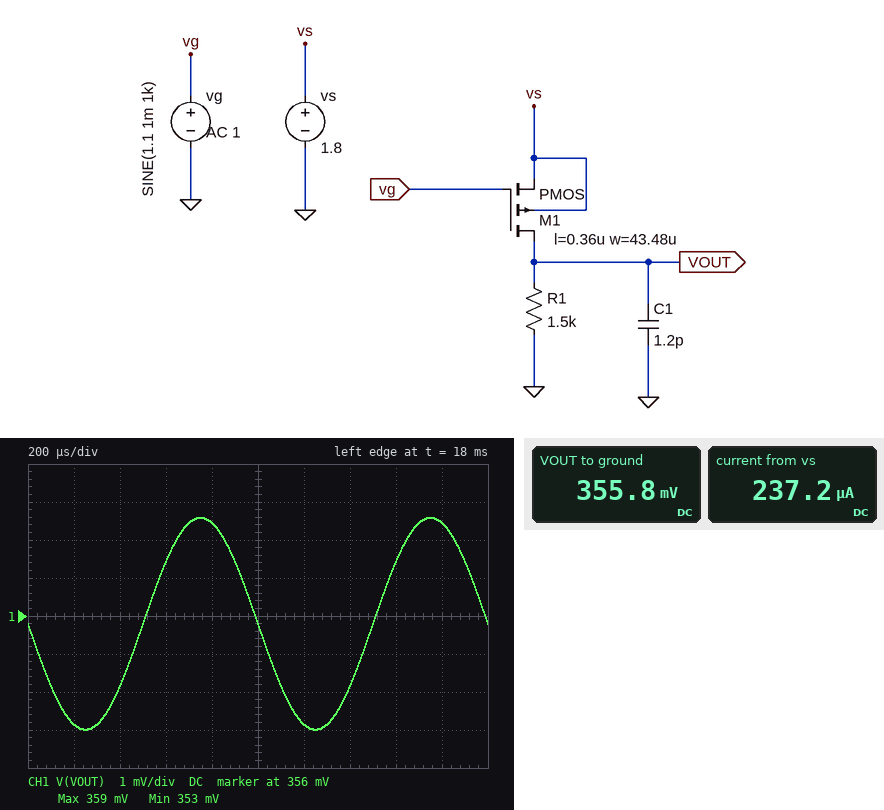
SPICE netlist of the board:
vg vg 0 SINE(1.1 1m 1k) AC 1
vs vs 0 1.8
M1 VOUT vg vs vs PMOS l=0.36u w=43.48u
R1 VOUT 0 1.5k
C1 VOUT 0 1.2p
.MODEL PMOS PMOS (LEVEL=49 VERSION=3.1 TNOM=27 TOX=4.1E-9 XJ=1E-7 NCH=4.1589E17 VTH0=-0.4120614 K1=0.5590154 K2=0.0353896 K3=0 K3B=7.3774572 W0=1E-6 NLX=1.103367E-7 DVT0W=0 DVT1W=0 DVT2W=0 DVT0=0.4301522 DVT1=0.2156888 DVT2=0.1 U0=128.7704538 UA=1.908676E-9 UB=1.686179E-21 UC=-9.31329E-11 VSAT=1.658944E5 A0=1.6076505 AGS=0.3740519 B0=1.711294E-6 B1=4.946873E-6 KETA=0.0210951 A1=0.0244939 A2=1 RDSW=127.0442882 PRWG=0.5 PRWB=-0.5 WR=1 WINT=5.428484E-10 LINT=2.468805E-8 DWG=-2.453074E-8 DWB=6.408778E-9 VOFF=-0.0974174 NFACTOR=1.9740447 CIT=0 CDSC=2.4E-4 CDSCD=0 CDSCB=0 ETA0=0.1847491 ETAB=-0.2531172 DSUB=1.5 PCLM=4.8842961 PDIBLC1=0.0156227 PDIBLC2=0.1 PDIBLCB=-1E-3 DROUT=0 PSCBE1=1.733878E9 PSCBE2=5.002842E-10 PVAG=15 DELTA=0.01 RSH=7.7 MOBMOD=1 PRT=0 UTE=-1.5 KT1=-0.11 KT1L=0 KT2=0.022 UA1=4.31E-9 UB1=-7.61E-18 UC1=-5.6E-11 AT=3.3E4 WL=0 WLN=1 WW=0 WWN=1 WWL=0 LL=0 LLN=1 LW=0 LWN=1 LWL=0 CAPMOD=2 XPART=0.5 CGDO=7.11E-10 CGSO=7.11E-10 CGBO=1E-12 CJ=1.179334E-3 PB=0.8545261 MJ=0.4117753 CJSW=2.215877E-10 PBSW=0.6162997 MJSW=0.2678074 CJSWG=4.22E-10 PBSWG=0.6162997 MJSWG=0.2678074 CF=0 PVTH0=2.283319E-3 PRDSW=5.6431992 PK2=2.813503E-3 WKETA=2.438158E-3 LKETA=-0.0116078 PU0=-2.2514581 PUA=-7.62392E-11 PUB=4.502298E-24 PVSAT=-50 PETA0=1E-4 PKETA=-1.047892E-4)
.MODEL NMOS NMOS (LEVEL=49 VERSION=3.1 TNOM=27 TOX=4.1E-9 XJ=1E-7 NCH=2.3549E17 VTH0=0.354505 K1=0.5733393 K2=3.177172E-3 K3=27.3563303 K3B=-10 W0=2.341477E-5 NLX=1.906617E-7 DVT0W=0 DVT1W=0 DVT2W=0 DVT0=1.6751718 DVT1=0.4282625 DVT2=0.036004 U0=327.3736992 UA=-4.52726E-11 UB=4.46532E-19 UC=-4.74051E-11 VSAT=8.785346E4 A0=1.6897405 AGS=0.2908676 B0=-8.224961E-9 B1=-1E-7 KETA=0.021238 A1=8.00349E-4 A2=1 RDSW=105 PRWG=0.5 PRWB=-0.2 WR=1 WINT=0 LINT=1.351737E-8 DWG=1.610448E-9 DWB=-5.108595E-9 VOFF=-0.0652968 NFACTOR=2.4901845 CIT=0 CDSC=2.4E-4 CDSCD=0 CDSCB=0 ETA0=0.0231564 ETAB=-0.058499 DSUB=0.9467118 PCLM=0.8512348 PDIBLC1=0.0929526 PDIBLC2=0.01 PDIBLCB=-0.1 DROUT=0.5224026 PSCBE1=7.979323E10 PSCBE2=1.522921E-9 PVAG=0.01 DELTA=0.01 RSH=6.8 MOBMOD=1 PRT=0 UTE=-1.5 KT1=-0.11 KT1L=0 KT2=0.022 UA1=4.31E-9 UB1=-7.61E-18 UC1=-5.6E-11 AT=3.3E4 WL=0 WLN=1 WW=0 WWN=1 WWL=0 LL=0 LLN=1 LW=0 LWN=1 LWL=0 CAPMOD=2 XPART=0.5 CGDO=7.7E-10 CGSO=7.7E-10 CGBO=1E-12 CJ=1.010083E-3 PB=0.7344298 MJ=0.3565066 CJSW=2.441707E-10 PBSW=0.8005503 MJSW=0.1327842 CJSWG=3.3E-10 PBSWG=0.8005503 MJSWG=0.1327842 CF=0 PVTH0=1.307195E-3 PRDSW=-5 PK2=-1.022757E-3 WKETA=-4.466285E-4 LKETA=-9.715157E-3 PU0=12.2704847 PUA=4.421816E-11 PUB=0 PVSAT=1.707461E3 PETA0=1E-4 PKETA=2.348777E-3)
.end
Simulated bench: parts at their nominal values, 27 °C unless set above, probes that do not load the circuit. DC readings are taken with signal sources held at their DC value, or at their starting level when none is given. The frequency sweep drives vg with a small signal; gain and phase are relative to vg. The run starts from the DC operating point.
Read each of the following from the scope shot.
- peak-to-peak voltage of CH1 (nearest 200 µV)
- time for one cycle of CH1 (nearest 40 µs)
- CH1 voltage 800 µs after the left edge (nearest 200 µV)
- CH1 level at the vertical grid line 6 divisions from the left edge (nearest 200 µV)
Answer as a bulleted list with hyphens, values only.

- 5.6 mV
- 1.00 ms
- 358.4 mV
- 353.2 mV
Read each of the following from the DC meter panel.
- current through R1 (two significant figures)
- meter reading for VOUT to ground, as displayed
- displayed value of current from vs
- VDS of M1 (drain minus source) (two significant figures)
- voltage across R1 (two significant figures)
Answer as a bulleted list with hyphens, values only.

- 240 µA
- 355.8 mV
- 237.2 µA
- -1.4 V
- 360 mV
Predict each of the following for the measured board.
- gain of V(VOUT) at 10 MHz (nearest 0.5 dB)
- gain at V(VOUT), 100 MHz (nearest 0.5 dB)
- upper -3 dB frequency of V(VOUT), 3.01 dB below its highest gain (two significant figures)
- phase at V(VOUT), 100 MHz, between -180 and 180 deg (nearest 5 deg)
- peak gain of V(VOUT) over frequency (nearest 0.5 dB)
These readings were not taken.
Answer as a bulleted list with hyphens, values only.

- 9.0 dB
- 5.5 dB
- 88 MHz
- 130 deg
- 9.0 dB
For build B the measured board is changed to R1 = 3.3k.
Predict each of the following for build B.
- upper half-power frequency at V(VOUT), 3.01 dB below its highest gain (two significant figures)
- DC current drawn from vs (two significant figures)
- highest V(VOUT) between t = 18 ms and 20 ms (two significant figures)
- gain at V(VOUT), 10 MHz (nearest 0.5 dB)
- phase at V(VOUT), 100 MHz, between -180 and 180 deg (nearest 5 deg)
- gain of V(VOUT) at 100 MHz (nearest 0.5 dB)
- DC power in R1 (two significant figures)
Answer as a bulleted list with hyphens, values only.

- 41 MHz
- 230 µA
- 760 mV
- 15.0 dB
- 110 deg
- 7.0 dB
- 170 µW
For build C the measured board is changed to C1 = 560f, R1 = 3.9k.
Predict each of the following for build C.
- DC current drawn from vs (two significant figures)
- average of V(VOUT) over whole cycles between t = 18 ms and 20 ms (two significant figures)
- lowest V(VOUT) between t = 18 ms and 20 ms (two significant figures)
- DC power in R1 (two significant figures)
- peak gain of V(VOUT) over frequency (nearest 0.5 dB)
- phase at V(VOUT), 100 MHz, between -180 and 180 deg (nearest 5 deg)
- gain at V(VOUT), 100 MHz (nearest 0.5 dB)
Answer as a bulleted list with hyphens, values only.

- 230 µA
- 890 mV
- 880 mV
- 200 µW
- 16.5 dB
- 125 deg
- 12.0 dB
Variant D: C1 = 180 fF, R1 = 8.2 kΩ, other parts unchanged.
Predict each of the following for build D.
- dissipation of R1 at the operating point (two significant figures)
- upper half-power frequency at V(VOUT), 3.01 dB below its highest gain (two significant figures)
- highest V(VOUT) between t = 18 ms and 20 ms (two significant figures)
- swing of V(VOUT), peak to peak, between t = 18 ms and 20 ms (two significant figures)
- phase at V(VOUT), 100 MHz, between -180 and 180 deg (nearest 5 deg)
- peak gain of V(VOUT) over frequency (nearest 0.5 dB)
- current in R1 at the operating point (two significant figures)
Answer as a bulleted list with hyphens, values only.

- 320 µW
- 320 MHz
- 1.6 V
- 6.1 mV
- 160 deg
- 9.5 dB
- 200 µA
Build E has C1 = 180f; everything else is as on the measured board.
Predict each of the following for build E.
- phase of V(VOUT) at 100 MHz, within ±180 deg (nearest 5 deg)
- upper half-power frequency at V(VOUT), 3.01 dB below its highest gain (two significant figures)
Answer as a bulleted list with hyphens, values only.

- 165 deg
- 490 MHz
